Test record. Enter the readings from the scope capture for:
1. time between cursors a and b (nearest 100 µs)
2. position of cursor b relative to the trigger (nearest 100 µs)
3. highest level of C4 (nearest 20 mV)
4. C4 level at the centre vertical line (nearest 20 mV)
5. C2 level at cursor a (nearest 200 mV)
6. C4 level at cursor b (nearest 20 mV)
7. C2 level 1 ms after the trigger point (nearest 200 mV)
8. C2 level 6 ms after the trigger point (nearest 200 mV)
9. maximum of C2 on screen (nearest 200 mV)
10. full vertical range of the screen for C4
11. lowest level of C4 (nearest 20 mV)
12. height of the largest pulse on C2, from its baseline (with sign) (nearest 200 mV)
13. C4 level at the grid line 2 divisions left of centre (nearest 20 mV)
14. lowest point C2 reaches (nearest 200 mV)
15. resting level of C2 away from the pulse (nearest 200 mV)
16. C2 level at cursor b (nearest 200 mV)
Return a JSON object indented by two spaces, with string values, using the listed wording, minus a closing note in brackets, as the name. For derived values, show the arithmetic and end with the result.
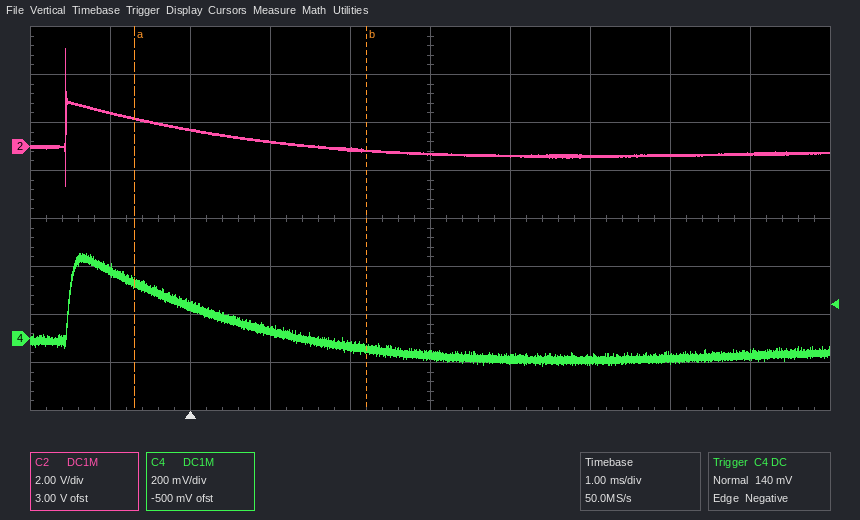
{
  "time between cursors a and b": "2.9 ms",
  "position of cursor b relative to the trigger": "+2.2 ms",
  "highest level of C4": "360 mV",
  "C4 level at the centre vertical line": "-60 mV",
  "C2 level at cursor a": "1.2 V",
  "C4 level at cursor b": "-40 mV",
  "C2 level 1 ms after the trigger point": "200 mV",
  "C2 level 6 ms after the trigger point": "-400 mV",
  "maximum of C2 on screen": "4.0 V",
  "full vertical range of the screen for C4": "1.6 V",
  "lowest level of C4": "-120 mV",
  "height of the largest pulse on C2, from its baseline (with sign)": "4.0 V − (-400 mV) = +4.4 V",
  "C4 level at the grid line 2 divisions left of centre": "40 mV",
  "lowest point C2 reaches": "-1.6 V",
  "resting level of C2 away from the pulse": "-400 mV",
  "C2 level at cursor b": "-200 mV"
}
